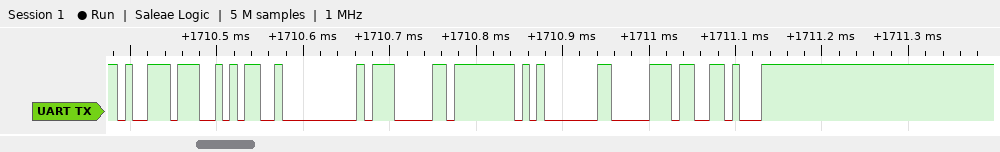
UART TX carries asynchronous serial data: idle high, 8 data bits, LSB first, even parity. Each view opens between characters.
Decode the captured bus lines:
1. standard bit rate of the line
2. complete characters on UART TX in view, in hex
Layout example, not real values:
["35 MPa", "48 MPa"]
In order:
["115200 baud", "B9, 6A, 00, 07, FF, 01, 70, 16"]
